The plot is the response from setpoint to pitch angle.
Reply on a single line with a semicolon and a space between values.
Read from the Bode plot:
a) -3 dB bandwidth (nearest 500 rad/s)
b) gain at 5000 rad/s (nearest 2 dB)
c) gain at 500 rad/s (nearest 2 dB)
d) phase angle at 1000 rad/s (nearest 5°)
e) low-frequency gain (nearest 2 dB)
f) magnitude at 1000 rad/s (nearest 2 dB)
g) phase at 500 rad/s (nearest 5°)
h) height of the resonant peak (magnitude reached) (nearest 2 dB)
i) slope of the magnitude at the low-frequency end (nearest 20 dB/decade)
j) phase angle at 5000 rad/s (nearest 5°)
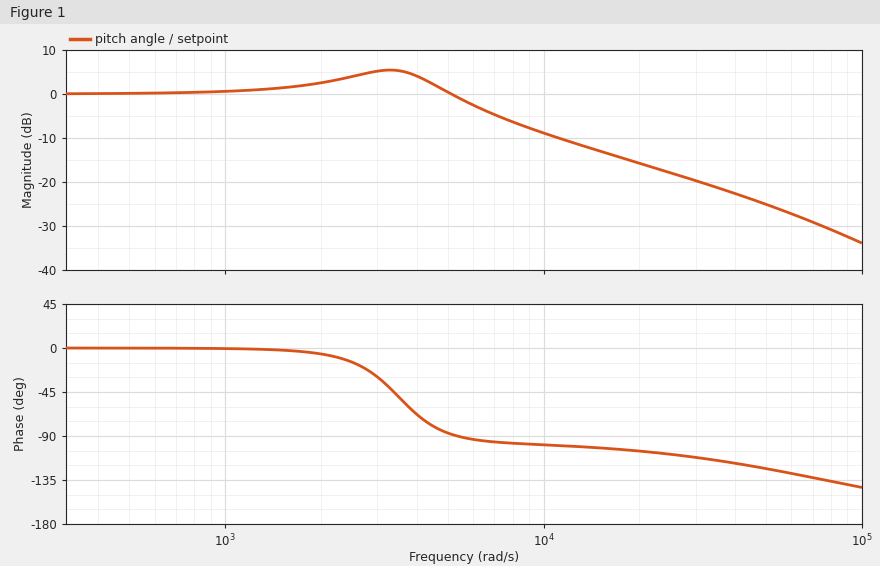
6000 rad/s; 0 dB; 0 dB; 0°; 0 dB; 0 dB; 0°; 6 dB; 0 dB/decade; -85°
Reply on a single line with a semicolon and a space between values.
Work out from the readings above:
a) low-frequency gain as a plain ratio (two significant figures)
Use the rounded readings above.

1.0
